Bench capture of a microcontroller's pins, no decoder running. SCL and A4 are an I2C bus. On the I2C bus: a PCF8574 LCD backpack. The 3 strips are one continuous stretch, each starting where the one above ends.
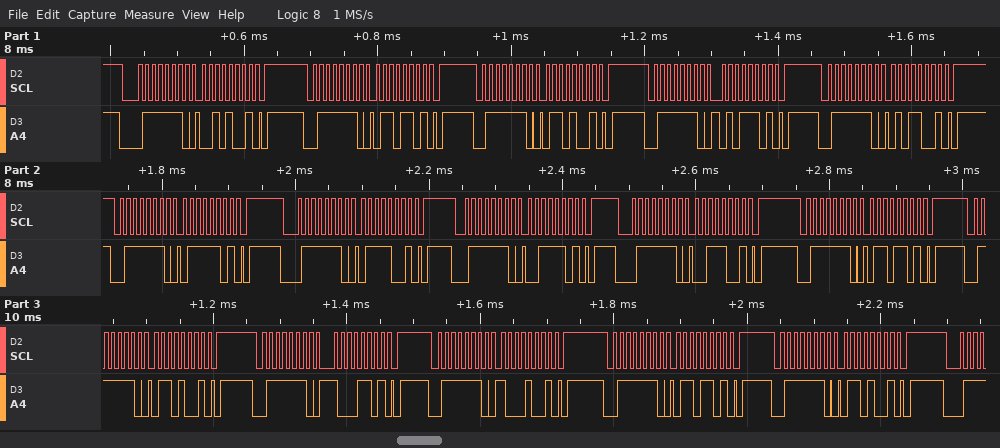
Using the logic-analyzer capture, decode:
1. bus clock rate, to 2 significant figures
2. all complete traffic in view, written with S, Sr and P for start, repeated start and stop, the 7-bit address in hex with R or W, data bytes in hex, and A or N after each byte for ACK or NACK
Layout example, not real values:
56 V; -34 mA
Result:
100 kHz; S 3FW A 29 A P S 3FW A 6D A P S 3FW A 69 A P S 3FW A 5D A P S 3FW A 59 A P S 3FW A 7D A P S 3FW A 79 A P S 3FW A 3D A P S 3FW A 39 A P S 3FW A 6D A P S 3FW A 69 A P S 3FW A 8D A P S 3FW A 89 A P S 3FW A 6D A P S 3FW A 69 A P
